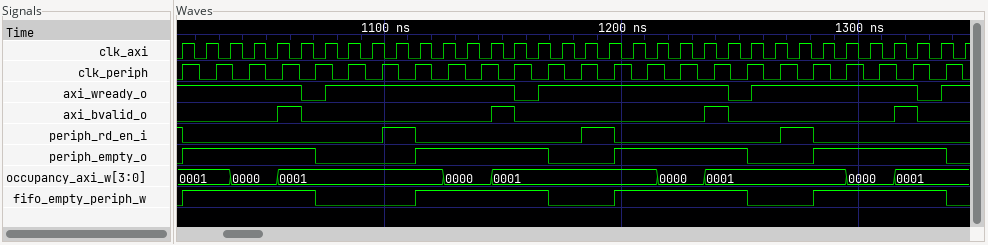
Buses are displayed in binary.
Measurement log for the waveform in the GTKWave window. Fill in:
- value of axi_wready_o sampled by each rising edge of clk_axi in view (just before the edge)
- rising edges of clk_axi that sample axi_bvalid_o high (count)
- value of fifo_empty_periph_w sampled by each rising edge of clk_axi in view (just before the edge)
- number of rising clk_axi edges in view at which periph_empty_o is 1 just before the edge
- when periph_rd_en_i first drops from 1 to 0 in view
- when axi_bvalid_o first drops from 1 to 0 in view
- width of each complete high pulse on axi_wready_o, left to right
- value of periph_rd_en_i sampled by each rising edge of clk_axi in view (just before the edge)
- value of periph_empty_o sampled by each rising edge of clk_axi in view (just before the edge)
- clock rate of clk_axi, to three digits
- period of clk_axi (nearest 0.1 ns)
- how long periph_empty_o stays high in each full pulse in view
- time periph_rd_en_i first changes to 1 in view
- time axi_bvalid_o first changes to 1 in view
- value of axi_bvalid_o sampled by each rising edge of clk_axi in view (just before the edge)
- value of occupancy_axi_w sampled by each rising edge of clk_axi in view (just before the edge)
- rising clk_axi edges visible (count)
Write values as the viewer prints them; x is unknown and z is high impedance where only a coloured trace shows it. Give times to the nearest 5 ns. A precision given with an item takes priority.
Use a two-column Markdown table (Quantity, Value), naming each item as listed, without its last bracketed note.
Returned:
| Quantity | Value |
|---|---|
| value of axi_wready_o sampled by each rising edge of clk_axi in view | 1 1 1 1 1 1 0 1 1 1 1 1 1 1 1 0 1 1 1 1 1 1 1 1 0 1 1 1 1 1 1 1 0 1 |
| rising edges of clk_axi that sample axi_bvalid_o high | 4 |
| value of fifo_empty_periph_w sampled by each rising edge of clk_axi in view | 0 1 1 1 1 1 0 0 0 0 1 1 1 1 1 1 0 0 0 1 1 1 1 1 0 0 0 1 1 1 1 1 1 0 |
| number of rising clk_axi edges in view at which periph_empty_o is 1 just before the edge | 22 |
| when periph_rd_en_i first drops from 1 to 0 in view | 1015 ns |
| when axi_bvalid_o first drops from 1 to 0 in view | 1065 ns |
| width of each complete high pulse on axi_wready_o, left to right | 80 ns, 80 ns, 70 ns |
| value of periph_rd_en_i sampled by each rising edge of clk_axi in view | 1 0 0 0 0 0 0 0 0 1 0 0 0 0 0 0 0 1 1 0 0 0 0 0 0 0 1 0 0 0 0 0 0 0 |
| value of periph_empty_o sampled by each rising edge of clk_axi in view | 0 1 1 1 1 1 0 0 0 0 1 1 1 1 1 1 0 0 0 1 1 1 1 1 0 0 0 1 1 1 1 1 1 0 |
| clock rate of clk_axi, to three digits | 100 MHz |
| period of clk_axi | 10 ns |
| how long periph_empty_o stays high in each full pulse in view | 55 ns, 55 ns, 55 ns, 55 ns |
| time periph_rd_en_i first changes to 1 in view | 1100 ns |
| time axi_bvalid_o first changes to 1 in view | 1055 ns |
| value of axi_bvalid_o sampled by each rising edge of clk_axi in view | 0 0 0 0 0 1 0 0 0 0 0 0 0 0 1 0 0 0 0 0 0 0 0 1 0 0 0 0 0 0 0 1 0 0 |
| value of occupancy_axi_w sampled by each rising edge of clk_axi in view | 0001, 0001, 0001, 0000, 0000, 0001, 0001, 0001, 0001, 0001, 0001, 0001, 0000, 0000, 0001, 0001, 0001, 0001, 0001, 0001, 0001, 0000, 0000, 0001, 0001, 0001, 0001, 0001, 0001, 0000, 0000, 0001, 0001, 0001 |
| rising clk_axi edges visible | 34 |
